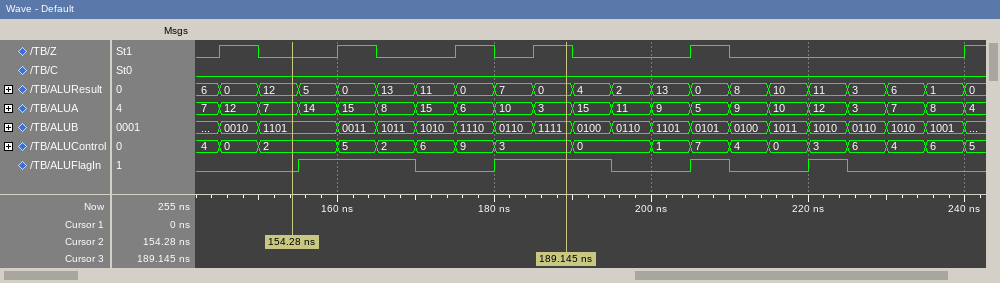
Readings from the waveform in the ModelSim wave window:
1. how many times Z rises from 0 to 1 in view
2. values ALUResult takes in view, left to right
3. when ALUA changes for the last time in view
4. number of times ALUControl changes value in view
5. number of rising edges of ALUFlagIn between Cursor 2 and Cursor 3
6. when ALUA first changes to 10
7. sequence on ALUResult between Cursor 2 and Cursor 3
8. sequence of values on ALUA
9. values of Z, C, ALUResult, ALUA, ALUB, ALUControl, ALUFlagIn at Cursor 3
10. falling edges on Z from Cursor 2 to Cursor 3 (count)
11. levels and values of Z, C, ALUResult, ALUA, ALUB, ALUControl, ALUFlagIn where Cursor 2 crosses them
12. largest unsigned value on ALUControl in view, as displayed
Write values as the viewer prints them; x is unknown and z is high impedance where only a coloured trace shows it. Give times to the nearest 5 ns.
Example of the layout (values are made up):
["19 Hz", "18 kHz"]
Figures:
["6", "6, 0, 12, 5, 0, 13, 11, 0, 7, 0, 4, 2, 13, 0, 8, 10, 11, 3, 6, 1, 0", "240 ns", "17", "2", "180 ns", "12, 5, 0, 13, 11, 0, 7, 0", "7, 12, 7, 14, 15, 8, 15, 6, 10, 3, 15, 11, 9, 5, 9, 10, 12, 3, 7, 8, 4", "Z=1, C=0, ALUResult=0, ALUA=3, ALUB=1111, ALUControl=3, ALUFlagIn=1", "2", "Z=0, C=0, ALUResult=12, ALUA=7, ALUB=1101, ALUControl=2, ALUFlagIn=0", "9"]
